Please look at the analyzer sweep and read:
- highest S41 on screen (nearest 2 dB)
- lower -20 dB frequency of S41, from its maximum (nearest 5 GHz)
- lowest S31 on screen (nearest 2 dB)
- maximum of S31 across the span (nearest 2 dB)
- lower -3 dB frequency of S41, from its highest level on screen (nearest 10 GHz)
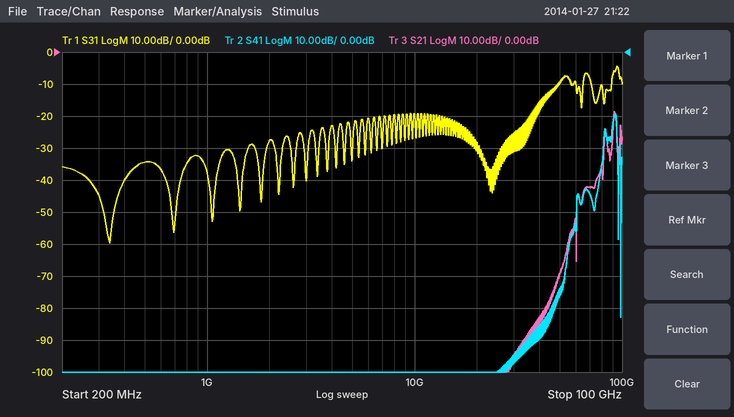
-20 dB
80 GHz
-60 dB
-4 dB
90 GHz
